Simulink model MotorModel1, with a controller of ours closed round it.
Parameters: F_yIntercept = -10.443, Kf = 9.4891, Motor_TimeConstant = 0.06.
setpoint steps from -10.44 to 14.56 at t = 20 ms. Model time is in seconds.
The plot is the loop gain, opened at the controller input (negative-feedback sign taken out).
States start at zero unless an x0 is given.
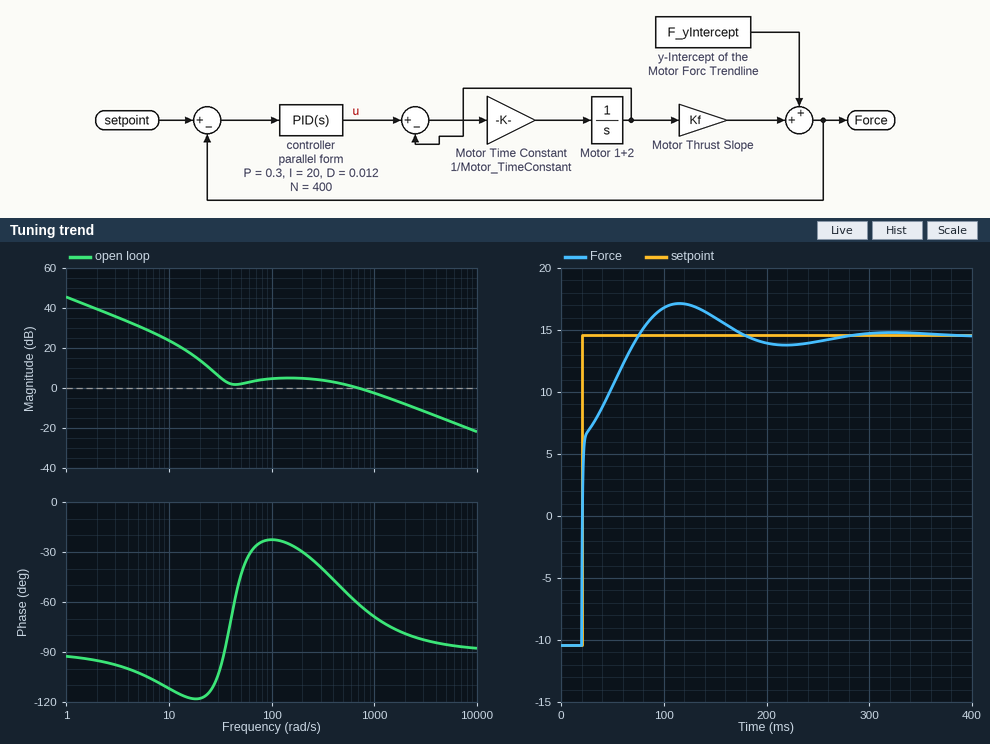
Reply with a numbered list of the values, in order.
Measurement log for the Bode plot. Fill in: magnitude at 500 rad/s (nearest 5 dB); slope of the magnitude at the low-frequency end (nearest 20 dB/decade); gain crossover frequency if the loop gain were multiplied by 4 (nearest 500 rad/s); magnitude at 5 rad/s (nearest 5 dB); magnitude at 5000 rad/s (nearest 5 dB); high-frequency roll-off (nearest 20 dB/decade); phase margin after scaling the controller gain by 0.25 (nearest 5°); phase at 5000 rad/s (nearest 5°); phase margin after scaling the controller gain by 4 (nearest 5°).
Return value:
1. 0 dB
2. -20 dB/decade
3. 3000 rad/s
4. 30 dB
5. -15 dB
6. -20 dB/decade
7. 65°
8. -85°
9. 95°
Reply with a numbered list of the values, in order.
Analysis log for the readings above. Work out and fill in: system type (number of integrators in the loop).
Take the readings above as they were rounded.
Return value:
1. 1
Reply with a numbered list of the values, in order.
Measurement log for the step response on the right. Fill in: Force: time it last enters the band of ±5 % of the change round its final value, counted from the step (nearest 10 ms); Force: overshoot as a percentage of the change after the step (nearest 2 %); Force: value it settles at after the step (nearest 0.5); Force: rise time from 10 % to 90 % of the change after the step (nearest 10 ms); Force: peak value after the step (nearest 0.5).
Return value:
1. 130 ms
2. 10 %
3. 14.5
4. 40 ms
5. 17.0
